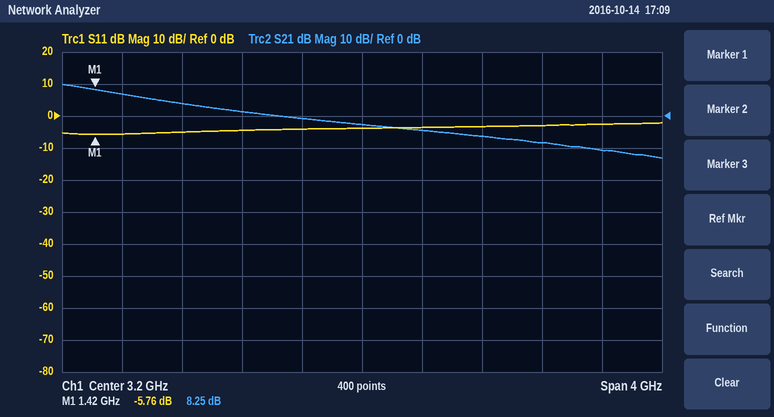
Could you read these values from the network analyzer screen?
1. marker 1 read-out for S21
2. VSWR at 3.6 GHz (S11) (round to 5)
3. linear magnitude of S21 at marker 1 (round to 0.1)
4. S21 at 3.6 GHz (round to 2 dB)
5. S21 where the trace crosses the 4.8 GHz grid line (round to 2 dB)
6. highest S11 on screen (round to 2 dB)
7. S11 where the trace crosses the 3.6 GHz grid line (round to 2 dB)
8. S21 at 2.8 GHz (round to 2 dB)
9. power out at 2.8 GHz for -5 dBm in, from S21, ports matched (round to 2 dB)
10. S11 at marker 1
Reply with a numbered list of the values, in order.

1. 8.25 dB
2. 5
3. 2.6
4. -4 dB
5. -10 dB
6. -2 dB
7. -4 dB
8. 0 dB
9. -6 dBm
10. -5.76 dB
